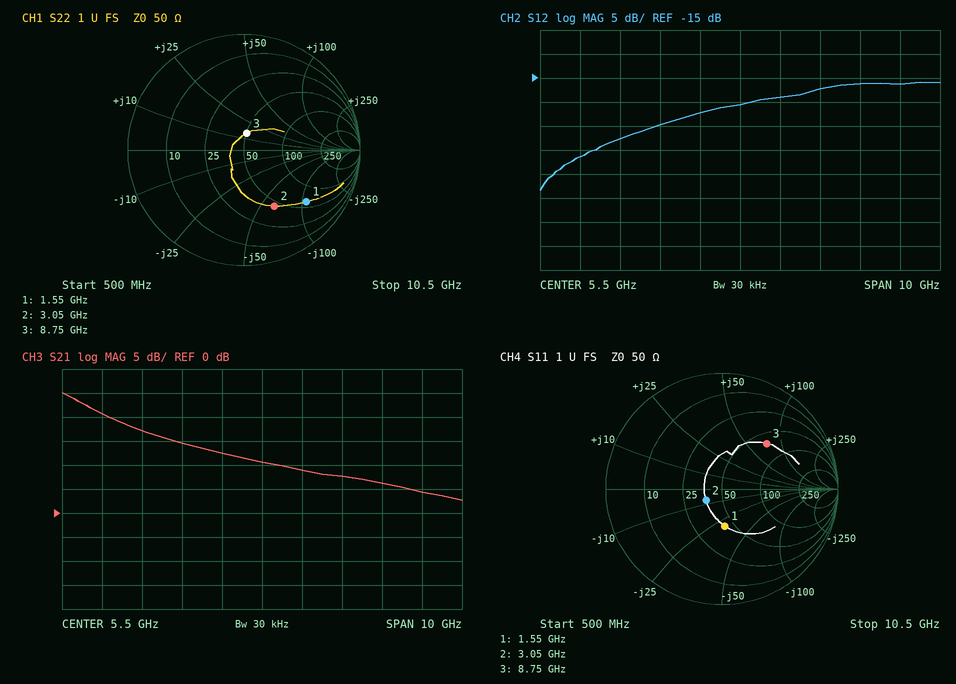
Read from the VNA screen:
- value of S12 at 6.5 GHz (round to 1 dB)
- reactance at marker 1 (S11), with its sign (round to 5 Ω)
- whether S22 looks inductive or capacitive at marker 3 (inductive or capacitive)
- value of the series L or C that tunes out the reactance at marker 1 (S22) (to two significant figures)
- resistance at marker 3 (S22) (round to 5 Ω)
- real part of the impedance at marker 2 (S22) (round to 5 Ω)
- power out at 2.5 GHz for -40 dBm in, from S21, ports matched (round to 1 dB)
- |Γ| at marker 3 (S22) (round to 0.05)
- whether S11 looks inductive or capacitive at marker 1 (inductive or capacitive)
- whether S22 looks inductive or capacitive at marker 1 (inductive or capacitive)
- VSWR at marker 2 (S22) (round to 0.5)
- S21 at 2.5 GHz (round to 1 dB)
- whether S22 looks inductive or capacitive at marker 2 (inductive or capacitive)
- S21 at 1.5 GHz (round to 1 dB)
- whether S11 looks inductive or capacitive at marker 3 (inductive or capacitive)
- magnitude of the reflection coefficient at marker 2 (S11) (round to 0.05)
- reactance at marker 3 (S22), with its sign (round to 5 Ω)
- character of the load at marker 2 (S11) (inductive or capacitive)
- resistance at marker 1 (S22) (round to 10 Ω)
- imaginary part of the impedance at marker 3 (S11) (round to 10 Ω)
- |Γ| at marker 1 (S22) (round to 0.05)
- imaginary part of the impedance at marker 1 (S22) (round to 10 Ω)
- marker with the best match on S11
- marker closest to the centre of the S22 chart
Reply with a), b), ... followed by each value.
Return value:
a) -19 dB
b) -30 Ω
c) inductive
d) 11 nH
e) 50 Ω
f) 45 Ω
g) -23 dBm
h) 0.15
i) capacitive
j) capacitive
k) 3.5
l) 17 dB
m) capacitive
n) 21 dB
o) inductive
p) 0.15
q) +15 Ω
r) capacitive
s) 60 Ω
t) +70 Ω
u) 0.70
v) -110 Ω
w) marker 2
x) marker 3
